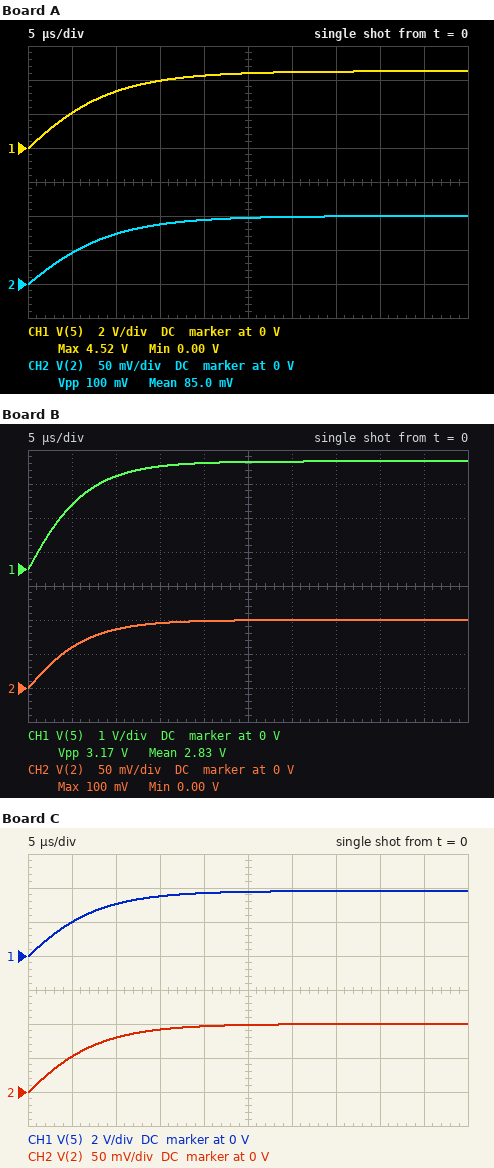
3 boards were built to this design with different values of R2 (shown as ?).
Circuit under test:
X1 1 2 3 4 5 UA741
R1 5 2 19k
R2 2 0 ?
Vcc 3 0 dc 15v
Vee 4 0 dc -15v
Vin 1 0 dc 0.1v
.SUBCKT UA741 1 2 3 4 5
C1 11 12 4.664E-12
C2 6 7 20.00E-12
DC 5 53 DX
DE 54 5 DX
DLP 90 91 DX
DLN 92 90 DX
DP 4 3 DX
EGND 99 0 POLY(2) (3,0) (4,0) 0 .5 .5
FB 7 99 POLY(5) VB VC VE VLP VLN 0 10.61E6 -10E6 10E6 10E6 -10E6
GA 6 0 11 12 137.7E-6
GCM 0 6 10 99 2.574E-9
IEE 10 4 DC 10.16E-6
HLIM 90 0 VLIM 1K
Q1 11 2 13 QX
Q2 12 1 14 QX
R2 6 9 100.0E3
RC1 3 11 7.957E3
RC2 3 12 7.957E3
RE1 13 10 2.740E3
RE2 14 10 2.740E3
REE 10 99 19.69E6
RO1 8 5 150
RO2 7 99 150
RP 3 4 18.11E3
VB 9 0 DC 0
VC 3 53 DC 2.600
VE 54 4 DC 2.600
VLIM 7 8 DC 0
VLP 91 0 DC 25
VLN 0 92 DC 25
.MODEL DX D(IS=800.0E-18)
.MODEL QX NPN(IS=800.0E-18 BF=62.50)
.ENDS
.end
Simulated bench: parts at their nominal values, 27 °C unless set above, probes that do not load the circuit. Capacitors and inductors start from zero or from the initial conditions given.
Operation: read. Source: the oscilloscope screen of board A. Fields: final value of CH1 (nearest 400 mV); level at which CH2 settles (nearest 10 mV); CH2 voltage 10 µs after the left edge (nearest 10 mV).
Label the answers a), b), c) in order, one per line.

a) 4.4 V
b) 100 mV
c) 70 mV
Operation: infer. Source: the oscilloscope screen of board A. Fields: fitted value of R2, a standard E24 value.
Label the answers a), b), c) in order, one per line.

a) 430 Ω
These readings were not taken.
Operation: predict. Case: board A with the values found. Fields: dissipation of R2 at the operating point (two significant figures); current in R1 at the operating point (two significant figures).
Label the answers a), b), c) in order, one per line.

a) 23 µW
b) 230 µA
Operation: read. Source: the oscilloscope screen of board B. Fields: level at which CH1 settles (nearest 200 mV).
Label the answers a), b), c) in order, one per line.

a) 3.2 V
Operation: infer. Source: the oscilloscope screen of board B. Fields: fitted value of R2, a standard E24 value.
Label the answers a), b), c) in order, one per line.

a) 620 Ω
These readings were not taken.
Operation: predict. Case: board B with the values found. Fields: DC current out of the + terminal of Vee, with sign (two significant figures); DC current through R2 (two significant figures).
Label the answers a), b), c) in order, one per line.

a) -1.7 mA
b) 160 µA
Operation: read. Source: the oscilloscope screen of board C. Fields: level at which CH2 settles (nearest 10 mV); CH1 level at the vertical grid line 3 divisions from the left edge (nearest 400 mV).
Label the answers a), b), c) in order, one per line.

a) 100 mV
b) 3.6 V
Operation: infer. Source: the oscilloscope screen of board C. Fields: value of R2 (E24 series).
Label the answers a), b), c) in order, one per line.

a) 510 Ω
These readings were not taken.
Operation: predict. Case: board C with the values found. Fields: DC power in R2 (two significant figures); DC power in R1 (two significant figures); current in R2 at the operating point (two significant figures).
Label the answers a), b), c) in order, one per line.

a) 20 µW
b) 730 µW
c) 200 µA
